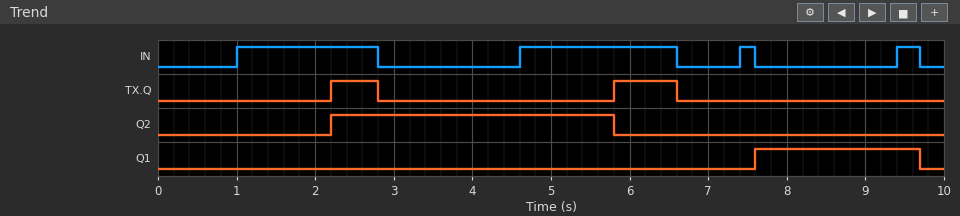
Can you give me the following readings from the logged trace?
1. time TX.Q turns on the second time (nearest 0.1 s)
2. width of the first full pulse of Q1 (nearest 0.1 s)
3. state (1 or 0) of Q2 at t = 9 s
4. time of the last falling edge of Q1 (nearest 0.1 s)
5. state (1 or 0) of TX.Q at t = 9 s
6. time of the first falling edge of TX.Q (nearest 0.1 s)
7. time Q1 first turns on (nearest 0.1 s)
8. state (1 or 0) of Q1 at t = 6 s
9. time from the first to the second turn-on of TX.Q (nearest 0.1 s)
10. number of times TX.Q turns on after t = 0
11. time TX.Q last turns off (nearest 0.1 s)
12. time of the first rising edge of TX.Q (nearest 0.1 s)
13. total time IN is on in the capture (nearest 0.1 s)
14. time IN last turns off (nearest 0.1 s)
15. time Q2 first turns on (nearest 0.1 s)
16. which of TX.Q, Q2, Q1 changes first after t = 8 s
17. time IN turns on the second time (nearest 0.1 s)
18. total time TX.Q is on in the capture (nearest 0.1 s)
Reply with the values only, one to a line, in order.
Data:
5.8 s
2.1 s
0
9.7 s
0
2.8 s
7.6 s
0
3.6 s
2
6.6 s
2.2 s
4.3 s
9.7 s
2.2 s
Q1
4.6 s
1.4 s
